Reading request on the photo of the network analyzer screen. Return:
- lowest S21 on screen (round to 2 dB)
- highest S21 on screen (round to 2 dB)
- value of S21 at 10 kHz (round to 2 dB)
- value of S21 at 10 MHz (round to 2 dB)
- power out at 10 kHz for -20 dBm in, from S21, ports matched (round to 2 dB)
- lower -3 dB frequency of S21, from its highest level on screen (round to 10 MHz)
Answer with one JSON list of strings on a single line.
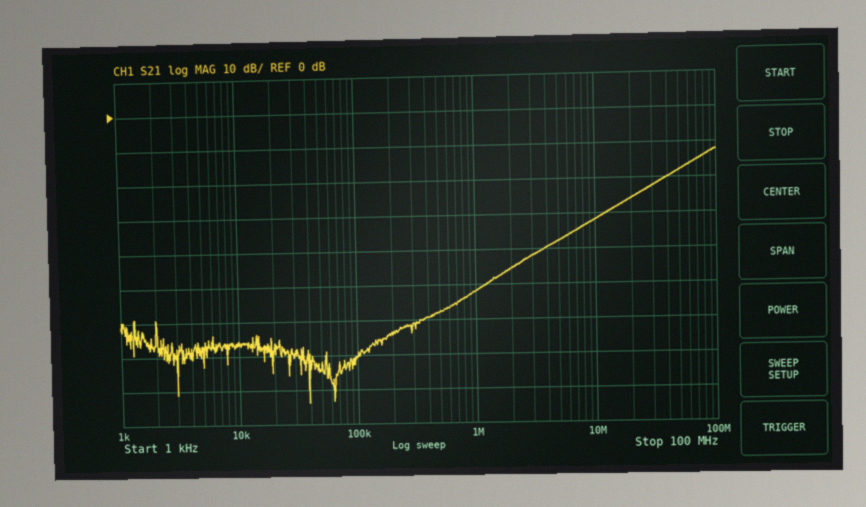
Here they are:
["-84 dB", "-12 dB", "-66 dB", "-32 dB", "-86 dBm", "70 MHz"]
